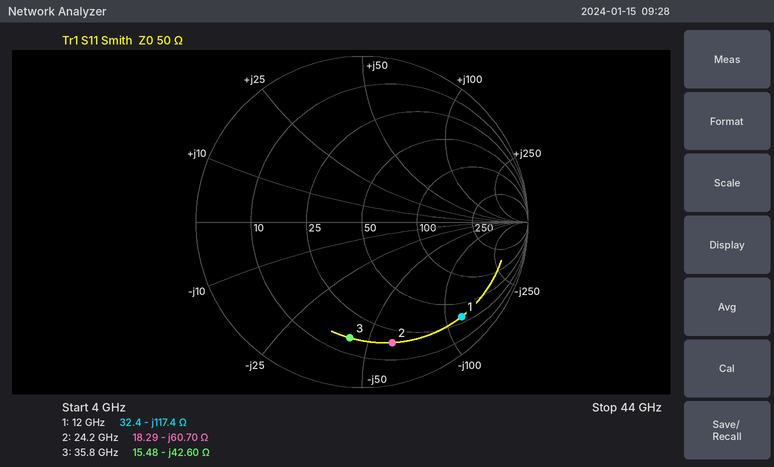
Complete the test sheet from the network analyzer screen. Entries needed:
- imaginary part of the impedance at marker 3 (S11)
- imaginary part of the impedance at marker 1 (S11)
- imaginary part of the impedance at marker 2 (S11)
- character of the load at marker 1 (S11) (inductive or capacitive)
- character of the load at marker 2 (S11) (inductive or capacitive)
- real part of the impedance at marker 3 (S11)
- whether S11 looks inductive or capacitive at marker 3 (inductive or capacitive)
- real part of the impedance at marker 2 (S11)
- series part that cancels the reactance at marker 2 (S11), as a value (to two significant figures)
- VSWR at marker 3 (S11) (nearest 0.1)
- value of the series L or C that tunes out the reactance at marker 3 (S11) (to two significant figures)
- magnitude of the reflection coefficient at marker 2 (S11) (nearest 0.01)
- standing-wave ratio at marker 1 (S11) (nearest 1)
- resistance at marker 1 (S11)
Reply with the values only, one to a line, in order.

-42.60 Ω
-117.4 Ω
-60.70 Ω
capacitive
capacitive
15.48 Ω
capacitive
18.29 Ω
400 pH
5.7
190 pH
0.75
11
32.4 Ω
